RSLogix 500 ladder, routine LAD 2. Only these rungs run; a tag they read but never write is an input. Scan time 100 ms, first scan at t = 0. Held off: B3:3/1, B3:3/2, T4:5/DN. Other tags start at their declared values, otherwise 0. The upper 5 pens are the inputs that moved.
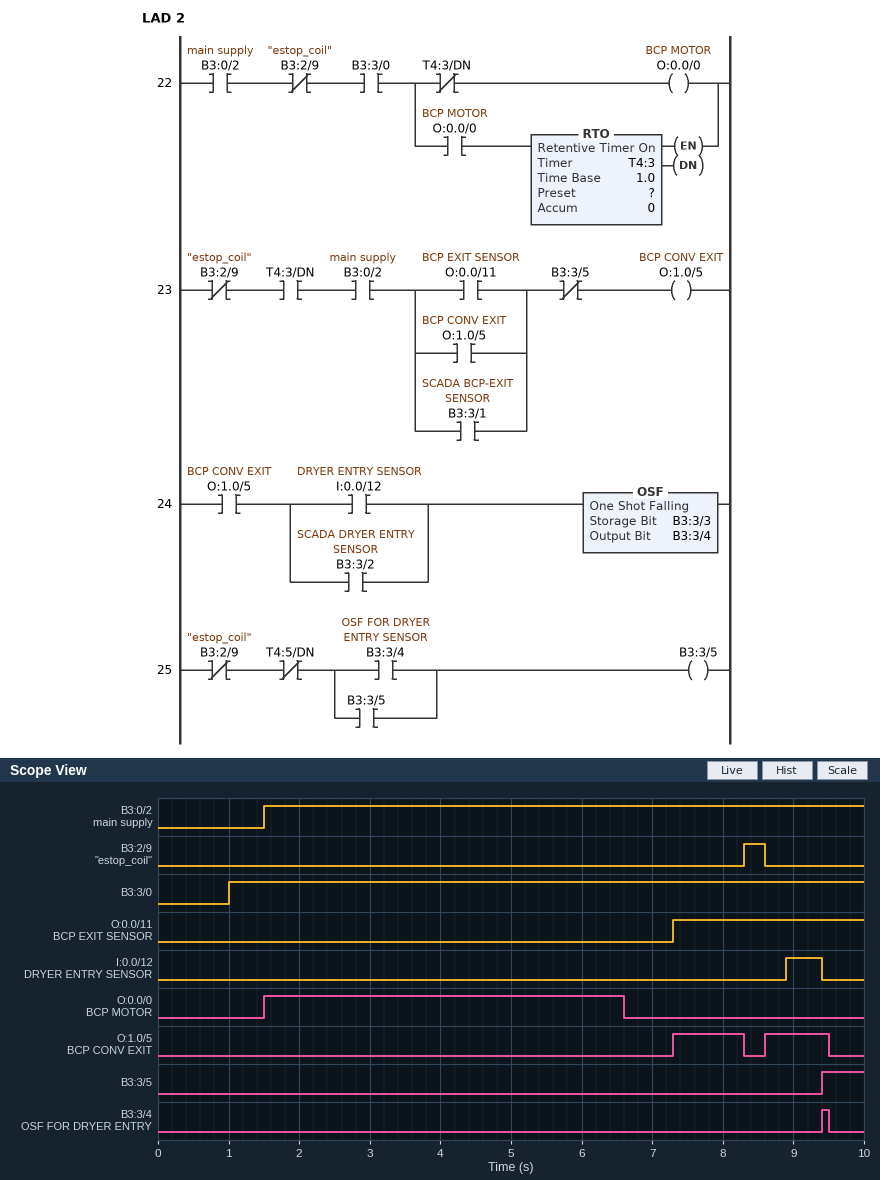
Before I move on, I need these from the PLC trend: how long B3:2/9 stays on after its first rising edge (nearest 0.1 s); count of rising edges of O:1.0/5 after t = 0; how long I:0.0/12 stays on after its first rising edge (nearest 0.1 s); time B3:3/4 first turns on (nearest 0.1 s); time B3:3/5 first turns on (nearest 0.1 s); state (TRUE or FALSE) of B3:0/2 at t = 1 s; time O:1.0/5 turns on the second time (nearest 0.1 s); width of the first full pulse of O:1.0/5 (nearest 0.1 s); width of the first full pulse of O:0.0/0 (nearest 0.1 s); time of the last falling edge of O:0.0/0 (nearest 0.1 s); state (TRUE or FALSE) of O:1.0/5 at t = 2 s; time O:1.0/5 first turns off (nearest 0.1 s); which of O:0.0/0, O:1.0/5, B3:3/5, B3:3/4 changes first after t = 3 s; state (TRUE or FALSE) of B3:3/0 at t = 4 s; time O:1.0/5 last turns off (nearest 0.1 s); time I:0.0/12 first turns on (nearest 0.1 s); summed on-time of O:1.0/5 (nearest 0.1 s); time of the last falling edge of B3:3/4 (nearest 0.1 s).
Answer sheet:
0.3 s
2
0.5 s
9.4 s
9.4 s
FALSE
8.6 s
1.0 s
5.1 s
6.6 s
FALSE
8.3 s
O:0.0/0
TRUE
9.5 s
8.9 s
1.9 s
9.5 s
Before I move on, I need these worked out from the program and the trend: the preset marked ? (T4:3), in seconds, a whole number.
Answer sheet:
5 s
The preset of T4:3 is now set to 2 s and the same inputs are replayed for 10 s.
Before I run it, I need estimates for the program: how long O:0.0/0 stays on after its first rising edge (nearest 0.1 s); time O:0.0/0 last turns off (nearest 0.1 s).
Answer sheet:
2.1 s
3.6 s
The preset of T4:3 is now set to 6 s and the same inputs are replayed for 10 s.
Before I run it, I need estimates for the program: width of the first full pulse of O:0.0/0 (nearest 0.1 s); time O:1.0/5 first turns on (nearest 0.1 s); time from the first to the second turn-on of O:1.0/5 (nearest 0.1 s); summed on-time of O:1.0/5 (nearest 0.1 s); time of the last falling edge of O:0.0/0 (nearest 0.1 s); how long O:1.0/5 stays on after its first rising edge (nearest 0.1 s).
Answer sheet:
6.1 s
7.5 s
1.1 s
1.7 s
7.6 s
0.8 s
